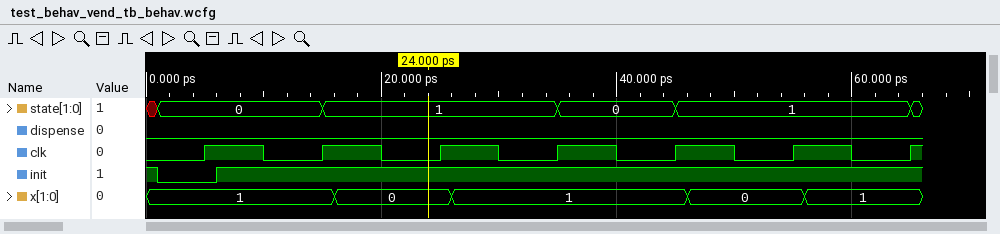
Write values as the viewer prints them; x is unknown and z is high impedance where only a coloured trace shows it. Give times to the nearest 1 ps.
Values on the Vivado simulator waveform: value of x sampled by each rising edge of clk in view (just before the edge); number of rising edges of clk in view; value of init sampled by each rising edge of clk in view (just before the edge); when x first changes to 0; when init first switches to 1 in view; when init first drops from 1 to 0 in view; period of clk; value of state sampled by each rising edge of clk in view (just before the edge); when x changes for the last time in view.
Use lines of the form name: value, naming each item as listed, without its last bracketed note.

value of x sampled by each rising edge of clk in view: 1, 1, 0, 1, 1, 0, 1
number of rising edges of clk in view: 7
value of init sampled by each rising edge of clk in view: 0 1 1 1 1 1 1
when x first changes to 0: 16 ps
when init first switches to 1 in view: 6 ps
when init first drops from 1 to 0 in view: 1 ps
period of clk: 10 ps
value of state sampled by each rising edge of clk in view: 0, 0, 1, 1, 0, 1, 1
when x changes for the last time in view: 56 ps
